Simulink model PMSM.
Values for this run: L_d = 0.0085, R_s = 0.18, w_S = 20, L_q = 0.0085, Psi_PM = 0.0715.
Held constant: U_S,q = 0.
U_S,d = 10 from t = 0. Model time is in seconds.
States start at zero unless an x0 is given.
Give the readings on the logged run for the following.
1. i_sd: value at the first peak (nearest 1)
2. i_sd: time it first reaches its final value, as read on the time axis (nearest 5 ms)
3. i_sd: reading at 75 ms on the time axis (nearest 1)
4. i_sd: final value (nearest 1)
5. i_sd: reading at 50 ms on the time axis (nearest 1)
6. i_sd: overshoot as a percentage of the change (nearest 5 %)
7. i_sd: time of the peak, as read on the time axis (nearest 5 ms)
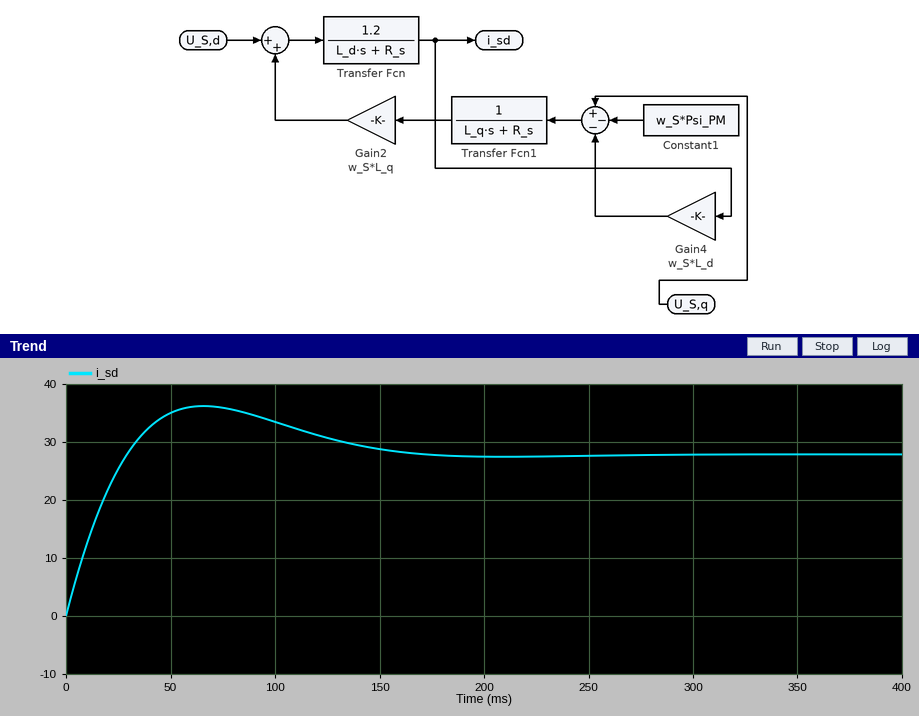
36
30 ms
36
28
35
30 %
65 ms
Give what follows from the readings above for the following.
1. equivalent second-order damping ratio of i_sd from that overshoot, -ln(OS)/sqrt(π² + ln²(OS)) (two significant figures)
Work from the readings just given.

0.36
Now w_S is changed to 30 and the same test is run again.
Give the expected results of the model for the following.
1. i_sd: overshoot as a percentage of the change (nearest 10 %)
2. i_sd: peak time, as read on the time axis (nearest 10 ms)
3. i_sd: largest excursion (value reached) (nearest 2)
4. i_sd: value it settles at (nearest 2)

90 %
40 ms
26
14
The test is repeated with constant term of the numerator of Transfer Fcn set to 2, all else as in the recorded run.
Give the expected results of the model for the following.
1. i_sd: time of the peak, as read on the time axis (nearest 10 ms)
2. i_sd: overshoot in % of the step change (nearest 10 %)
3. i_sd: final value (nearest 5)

50 ms
50 %
35
